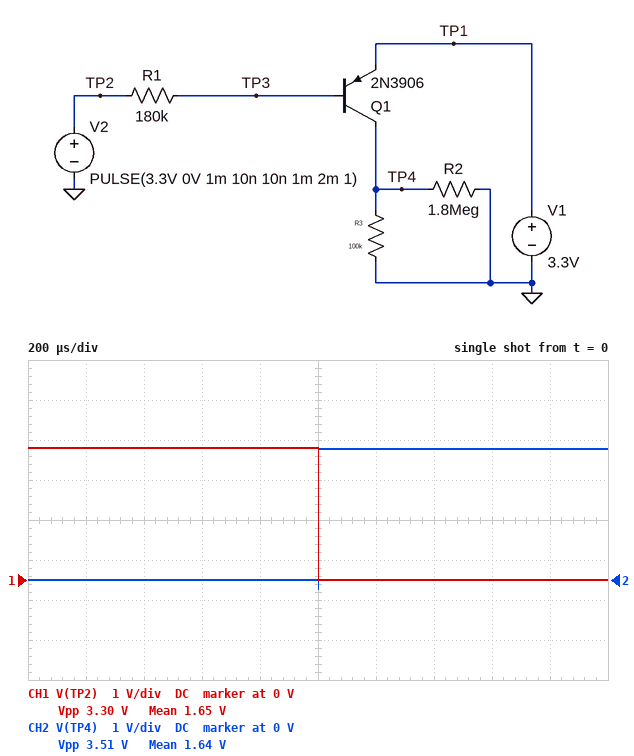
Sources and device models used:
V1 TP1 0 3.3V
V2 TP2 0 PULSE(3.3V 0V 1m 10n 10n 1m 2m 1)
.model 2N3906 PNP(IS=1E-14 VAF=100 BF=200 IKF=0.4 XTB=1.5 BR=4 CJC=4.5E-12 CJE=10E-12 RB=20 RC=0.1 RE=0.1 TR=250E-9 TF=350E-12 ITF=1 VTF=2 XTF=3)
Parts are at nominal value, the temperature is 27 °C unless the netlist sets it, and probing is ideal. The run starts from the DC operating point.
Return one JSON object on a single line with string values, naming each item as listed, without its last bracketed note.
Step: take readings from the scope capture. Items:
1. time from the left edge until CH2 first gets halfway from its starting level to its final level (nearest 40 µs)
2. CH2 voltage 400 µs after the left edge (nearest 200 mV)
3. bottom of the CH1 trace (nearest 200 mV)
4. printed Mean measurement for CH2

{"time from the left edge until CH2 first gets halfway from its starting level to its final level": "1.00 ms", "CH2 voltage 400 µs after the left edge": "0 V", "bottom of the CH1 trace": "0 V", "printed Mean measurement for CH2": "1.64 V"}
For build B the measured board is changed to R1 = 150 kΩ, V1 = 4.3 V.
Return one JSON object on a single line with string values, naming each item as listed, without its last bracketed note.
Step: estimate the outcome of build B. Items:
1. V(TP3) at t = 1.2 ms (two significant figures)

{"V(TP3) at t = 1.2 ms": "3.7 V"}
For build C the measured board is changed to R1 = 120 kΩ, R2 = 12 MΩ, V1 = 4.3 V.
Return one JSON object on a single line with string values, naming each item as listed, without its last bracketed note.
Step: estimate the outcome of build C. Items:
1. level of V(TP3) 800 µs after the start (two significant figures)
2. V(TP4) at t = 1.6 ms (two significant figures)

{"level of V(TP3) 800 µs after the start": "3.7 V", "V(TP4) at t = 1.6 ms": "4.3 V"}
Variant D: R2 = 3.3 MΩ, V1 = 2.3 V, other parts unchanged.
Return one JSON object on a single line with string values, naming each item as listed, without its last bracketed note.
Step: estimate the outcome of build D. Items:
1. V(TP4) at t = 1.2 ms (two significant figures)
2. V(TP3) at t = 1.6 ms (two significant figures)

{"V(TP4) at t = 1.2 ms": "2.3 V", "V(TP3) at t = 1.6 ms": "1.7 V"}
